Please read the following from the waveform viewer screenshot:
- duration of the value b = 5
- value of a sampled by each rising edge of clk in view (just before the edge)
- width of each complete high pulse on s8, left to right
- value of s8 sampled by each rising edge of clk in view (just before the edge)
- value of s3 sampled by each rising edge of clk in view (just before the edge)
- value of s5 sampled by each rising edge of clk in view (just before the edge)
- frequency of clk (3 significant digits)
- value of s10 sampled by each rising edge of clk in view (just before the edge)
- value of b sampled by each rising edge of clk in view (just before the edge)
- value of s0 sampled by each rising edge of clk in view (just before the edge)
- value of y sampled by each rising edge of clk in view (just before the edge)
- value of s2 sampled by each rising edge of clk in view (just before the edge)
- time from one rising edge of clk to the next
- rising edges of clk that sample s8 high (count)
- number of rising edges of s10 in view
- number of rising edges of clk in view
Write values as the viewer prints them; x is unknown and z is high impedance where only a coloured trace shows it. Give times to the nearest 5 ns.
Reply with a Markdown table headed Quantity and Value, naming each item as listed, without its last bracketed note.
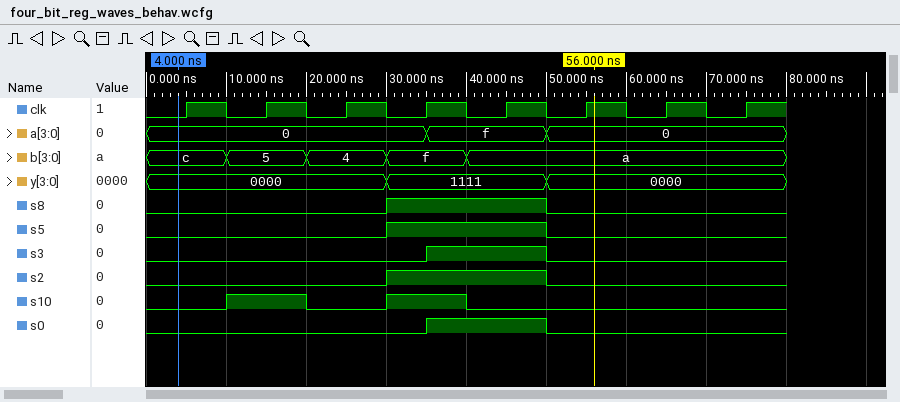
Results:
| Quantity | Value |
|---|---|
| duration of the value b = 5 | 10 ns |
| value of a sampled by each rising edge of clk in view | 0, 0, 0, 0, f, 0, 0, 0 |
| width of each complete high pulse on s8, left to right | 20 ns |
| value of s8 sampled by each rising edge of clk in view | 0 0 0 1 1 0 0 0 |
| value of s3 sampled by each rising edge of clk in view | 0 0 0 0 1 0 0 0 |
| value of s5 sampled by each rising edge of clk in view | 0 0 0 1 1 0 0 0 |
| frequency of clk | 100 MHz |
| value of s10 sampled by each rising edge of clk in view | 0 1 0 1 0 0 0 0 |
| value of b sampled by each rising edge of clk in view | c, 5, 4, f, a, a, a, a |
| value of s0 sampled by each rising edge of clk in view | 0 0 0 0 1 0 0 0 |
| value of y sampled by each rising edge of clk in view | 0000, 0000, 0000, 1111, 1111, 0000, 0000, 0000 |
| value of s2 sampled by each rising edge of clk in view | 0 0 0 1 1 0 0 0 |
| time from one rising edge of clk to the next | 10 ns |
| rising edges of clk that sample s8 high | 2 |
| number of rising edges of s10 in view | 2 |
| number of rising edges of clk in view | 8 |
